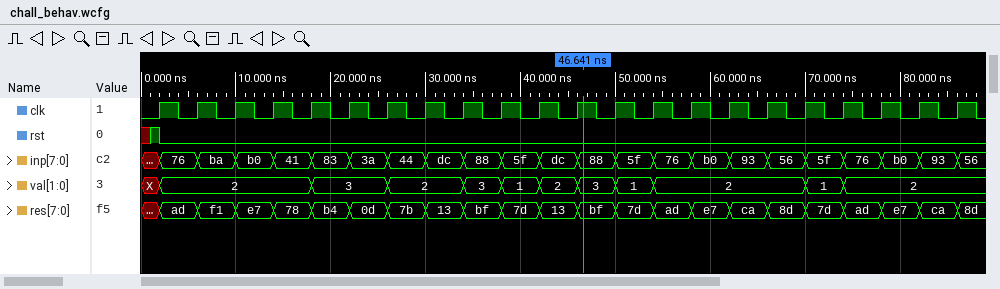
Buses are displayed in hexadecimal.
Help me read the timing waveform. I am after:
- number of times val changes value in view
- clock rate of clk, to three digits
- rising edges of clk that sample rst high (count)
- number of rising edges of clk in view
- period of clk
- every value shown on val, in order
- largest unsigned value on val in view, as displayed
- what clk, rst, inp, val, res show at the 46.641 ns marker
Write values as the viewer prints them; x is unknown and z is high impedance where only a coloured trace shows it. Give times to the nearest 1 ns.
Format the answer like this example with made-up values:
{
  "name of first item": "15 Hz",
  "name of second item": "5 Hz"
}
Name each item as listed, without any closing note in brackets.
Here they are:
{
  "number of times val changes value in view": "11",
  "clock rate of clk, to three digits": "250 MHz",
  "rising edges of clk that sample rst high": "1",
  "number of rising edges of clk in view": "22",
  "period of clk": "4 ns",
  "every value shown on val, in order": "X, 2, 3, 2, 3, 1, 2, 3, 1, 2, 1, 2",
  "largest unsigned value on val in view, as displayed": "3",
  "what clk, rst, inp, val, res show at the 46.641 ns marker": "clk=1, rst=0, inp=88, val=3, res=bf"
}
